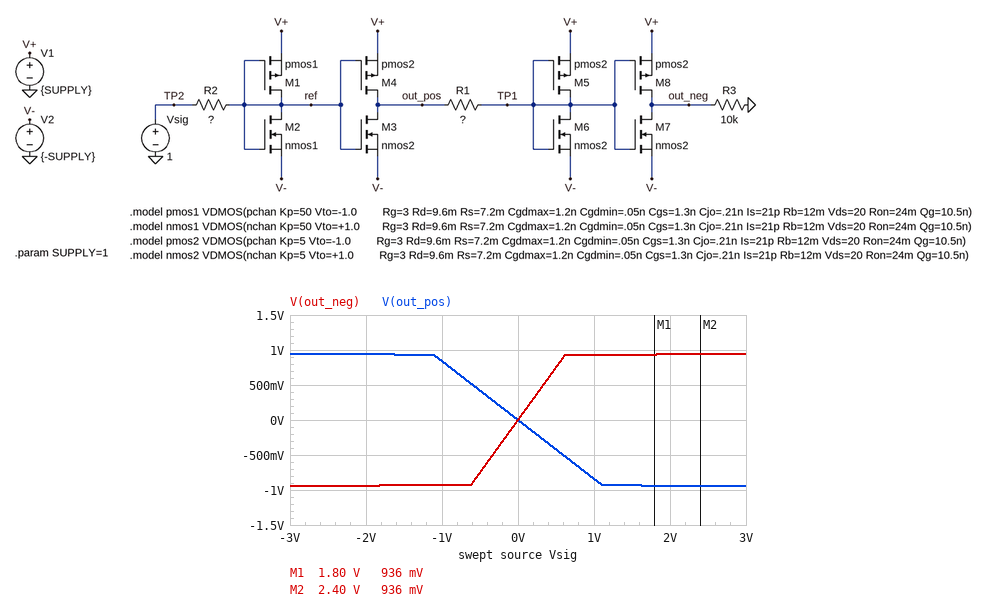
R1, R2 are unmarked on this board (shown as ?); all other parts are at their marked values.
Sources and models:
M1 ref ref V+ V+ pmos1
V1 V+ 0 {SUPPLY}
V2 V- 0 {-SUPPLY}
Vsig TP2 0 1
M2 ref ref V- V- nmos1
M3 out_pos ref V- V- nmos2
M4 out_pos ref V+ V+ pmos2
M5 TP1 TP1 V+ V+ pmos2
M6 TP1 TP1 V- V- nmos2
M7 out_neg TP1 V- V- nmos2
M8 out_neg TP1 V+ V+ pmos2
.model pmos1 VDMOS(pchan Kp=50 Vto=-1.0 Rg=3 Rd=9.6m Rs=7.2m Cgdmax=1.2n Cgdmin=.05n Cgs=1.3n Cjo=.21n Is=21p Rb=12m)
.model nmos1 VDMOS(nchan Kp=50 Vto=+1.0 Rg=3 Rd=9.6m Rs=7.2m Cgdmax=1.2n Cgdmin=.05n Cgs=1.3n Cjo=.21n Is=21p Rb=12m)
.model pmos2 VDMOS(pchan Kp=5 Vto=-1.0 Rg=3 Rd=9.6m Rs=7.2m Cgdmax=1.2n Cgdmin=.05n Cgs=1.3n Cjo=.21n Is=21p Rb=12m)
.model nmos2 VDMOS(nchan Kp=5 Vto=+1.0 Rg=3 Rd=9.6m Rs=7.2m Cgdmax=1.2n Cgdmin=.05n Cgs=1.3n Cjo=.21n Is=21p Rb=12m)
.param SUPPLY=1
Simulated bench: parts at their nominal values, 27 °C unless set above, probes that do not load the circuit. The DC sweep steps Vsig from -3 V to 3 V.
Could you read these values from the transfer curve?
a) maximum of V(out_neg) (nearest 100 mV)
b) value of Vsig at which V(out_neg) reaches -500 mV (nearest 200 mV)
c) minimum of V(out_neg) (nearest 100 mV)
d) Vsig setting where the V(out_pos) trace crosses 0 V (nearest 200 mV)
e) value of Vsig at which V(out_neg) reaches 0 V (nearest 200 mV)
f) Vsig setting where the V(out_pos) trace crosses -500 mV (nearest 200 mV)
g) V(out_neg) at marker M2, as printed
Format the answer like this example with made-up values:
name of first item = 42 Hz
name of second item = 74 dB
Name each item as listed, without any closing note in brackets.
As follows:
maximum of V(out_neg) = 900 mV
value of Vsig at which V(out_neg) reaches -500 mV = -400 mV
minimum of V(out_neg) = -900 mV
Vsig setting where the V(out_pos) trace crosses 0 V = 0 V
value of Vsig at which V(out_neg) reaches 0 V = 0 V
Vsig setting where the V(out_pos) trace crosses -500 mV = 600 mV
V(out_neg) at marker M2, as printed = 936 mV
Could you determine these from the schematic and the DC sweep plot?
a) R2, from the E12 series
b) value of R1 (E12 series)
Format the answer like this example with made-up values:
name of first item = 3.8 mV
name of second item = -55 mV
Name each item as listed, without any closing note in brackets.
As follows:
R2, from the E12 series = 680 Ω
value of R1 = 5.6 kΩ
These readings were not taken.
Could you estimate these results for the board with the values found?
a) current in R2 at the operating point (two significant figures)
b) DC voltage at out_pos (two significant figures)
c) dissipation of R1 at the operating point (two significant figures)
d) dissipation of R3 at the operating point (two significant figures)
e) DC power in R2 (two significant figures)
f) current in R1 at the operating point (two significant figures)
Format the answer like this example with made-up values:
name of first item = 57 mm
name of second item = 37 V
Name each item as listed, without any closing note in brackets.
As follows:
current in R2 at the operating point = 1.5 mA
DC voltage at out_pos = -840 mV
dissipation of R1 at the operating point = 130 µW
dissipation of R3 at the operating point = 87 µW
DC power in R2 = 1.5 mW
current in R1 at the operating point = 150 µA
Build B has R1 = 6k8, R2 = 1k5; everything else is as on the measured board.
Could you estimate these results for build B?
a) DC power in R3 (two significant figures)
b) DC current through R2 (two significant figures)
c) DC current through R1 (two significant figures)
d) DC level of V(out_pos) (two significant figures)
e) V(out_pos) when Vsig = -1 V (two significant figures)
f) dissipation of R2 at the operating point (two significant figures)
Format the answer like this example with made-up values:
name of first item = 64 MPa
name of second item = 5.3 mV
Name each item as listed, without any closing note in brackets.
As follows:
DC power in R3 = 46 µW
DC current through R2 = 670 µA
DC current through R1 = 68 µA
DC level of V(out_pos) = -460 mV
V(out_pos) when Vsig = -1 V = 460 mV
dissipation of R2 at the operating point = 670 µW
